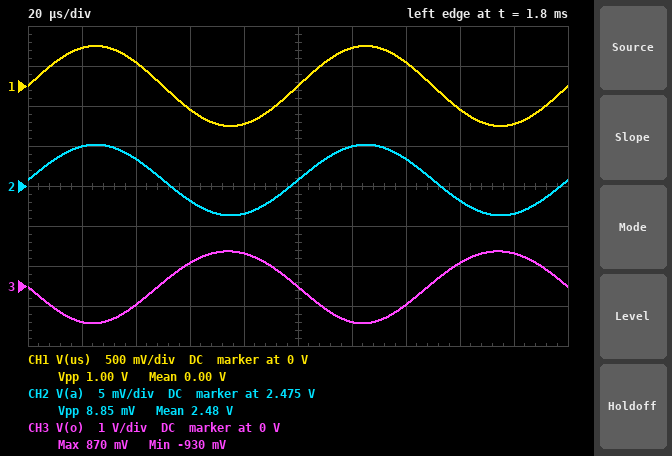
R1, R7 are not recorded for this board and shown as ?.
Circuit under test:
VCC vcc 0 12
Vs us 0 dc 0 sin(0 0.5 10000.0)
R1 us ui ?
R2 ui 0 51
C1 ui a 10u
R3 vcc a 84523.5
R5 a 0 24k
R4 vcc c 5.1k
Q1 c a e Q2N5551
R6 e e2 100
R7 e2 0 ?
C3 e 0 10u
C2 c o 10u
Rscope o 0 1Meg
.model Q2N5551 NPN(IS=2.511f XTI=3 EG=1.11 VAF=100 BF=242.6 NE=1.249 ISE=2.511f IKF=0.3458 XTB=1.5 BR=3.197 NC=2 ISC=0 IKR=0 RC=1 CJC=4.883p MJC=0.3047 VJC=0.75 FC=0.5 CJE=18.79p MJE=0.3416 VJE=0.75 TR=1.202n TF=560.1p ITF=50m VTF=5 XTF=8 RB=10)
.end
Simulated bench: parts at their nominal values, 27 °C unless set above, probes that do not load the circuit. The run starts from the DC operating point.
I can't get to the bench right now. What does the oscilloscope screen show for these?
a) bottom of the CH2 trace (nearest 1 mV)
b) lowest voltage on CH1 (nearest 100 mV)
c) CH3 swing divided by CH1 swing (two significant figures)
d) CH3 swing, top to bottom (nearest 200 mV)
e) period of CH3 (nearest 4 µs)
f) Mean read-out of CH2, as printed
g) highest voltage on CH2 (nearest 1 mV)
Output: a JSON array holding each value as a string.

["2.471 V", "-500 mV", "1.8", "1.8 V", "100 µs", "2.48 V", "2.480 V"]
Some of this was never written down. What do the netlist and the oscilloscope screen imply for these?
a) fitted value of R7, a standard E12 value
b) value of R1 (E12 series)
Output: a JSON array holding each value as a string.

["1.5 kΩ", "5.6 kΩ"]
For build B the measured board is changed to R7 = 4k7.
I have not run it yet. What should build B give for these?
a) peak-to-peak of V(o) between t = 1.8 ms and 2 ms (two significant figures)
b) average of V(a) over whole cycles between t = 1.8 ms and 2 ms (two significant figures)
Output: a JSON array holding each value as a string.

["680 mV", "2.6 V"]
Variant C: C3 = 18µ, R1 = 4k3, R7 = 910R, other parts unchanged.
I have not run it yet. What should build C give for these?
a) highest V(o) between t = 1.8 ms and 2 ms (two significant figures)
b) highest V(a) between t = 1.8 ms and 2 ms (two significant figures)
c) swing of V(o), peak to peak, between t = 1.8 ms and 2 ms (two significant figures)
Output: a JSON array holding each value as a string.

["1.6 V", "2.4 V", "3.3 V"]
